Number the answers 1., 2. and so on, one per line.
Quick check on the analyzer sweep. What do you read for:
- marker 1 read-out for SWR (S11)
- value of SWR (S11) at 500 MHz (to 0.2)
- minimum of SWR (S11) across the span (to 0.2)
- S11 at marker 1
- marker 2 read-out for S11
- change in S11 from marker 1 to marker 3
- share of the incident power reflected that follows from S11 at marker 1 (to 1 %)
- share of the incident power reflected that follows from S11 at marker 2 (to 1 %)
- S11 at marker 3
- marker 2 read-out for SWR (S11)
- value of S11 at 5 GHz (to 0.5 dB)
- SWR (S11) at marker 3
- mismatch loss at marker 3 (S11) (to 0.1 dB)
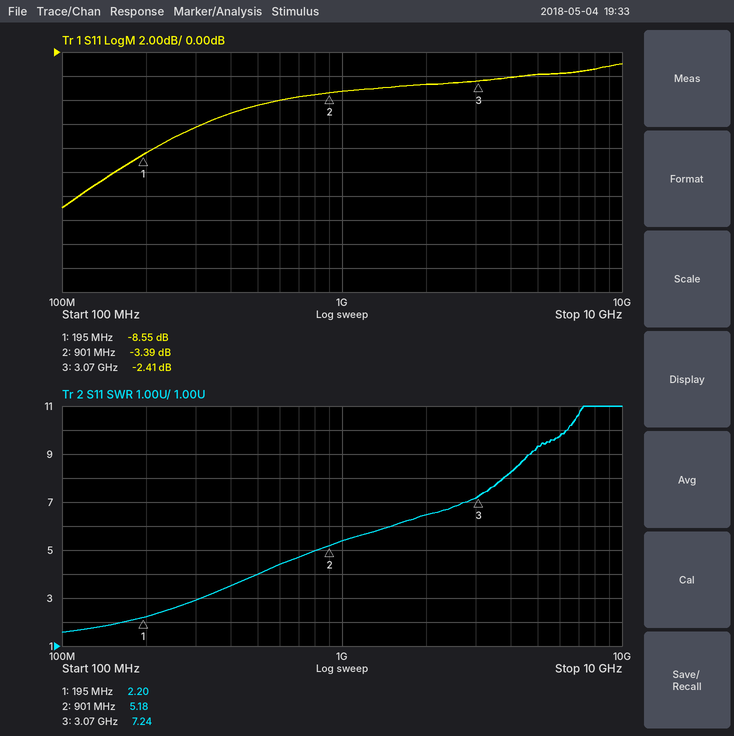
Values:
1. 2.20
2. 4.0
3. 1.6
4. -8.55 dB
5. -3.39 dB
6. 6.14 dB
7. 14 %
8. 46 %
9. -2.41 dB
10. 5.18
11. -2.0 dB
12. 7.24
13. 3.7 dB
